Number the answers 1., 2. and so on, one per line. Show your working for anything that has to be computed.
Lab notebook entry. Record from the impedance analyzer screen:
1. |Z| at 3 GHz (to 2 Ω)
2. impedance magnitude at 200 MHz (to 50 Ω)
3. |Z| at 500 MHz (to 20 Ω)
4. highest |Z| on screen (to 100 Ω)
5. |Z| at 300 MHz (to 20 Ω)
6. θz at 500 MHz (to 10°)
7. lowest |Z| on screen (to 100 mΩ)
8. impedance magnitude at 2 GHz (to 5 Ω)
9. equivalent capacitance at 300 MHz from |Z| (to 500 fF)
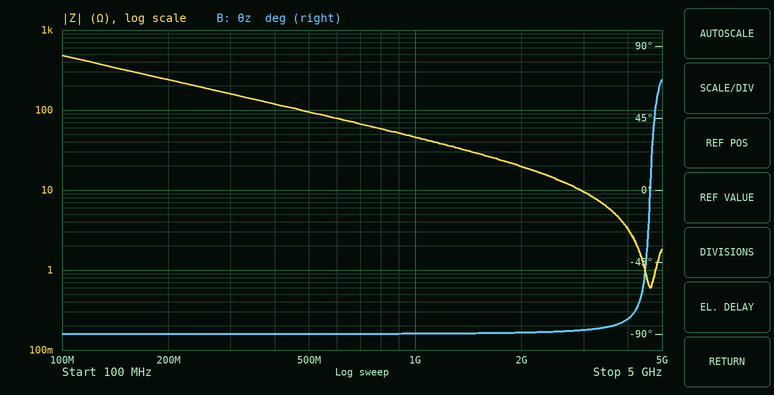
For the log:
1. 10 Ω
2. 250 Ω
3. 100 Ω
4. 500 Ω
5. 160 Ω
6. -90°
7. 600 mΩ
8. 20 Ω
9. C = 1/(2π × 300 MHz × 160 Ω) ≈ 3.32 pF, so 3.5 pF to the nearest 500 fF
